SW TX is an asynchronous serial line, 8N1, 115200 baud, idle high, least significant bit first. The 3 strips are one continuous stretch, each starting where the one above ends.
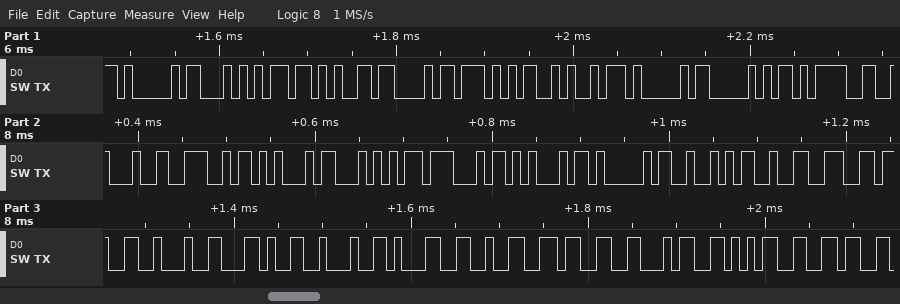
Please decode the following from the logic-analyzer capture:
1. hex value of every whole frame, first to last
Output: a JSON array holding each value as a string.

["41 54 2B 43 57 4A 41 50 3D 22 4E 45 54 47 45 41 52 32 36 22 2C 22 31 32 33 34 35 36"]
